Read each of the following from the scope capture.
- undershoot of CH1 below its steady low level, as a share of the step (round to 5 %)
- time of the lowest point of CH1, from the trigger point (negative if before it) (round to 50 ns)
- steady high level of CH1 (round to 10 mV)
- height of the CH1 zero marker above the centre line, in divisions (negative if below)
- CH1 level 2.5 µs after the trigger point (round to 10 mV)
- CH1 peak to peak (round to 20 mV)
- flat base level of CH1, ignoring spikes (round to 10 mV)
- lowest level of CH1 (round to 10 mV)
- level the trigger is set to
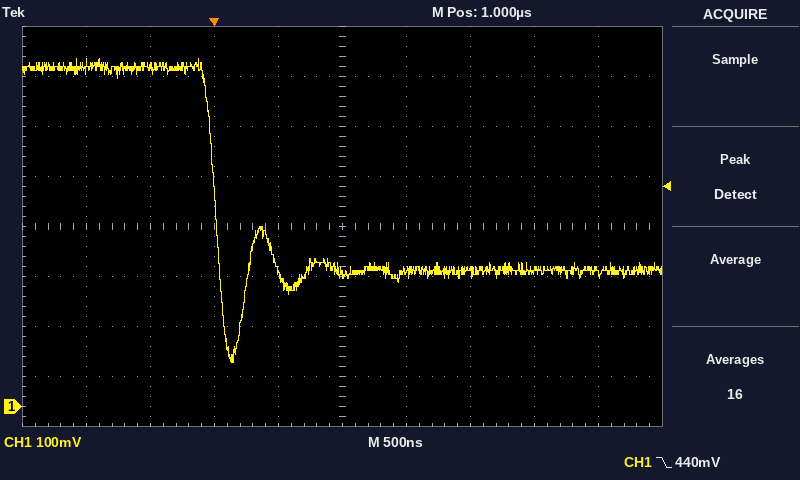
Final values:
45 %
+150 ns
680 mV
-3.6 div
270 mV
600 mV
270 mV
90 mV
440 mV
